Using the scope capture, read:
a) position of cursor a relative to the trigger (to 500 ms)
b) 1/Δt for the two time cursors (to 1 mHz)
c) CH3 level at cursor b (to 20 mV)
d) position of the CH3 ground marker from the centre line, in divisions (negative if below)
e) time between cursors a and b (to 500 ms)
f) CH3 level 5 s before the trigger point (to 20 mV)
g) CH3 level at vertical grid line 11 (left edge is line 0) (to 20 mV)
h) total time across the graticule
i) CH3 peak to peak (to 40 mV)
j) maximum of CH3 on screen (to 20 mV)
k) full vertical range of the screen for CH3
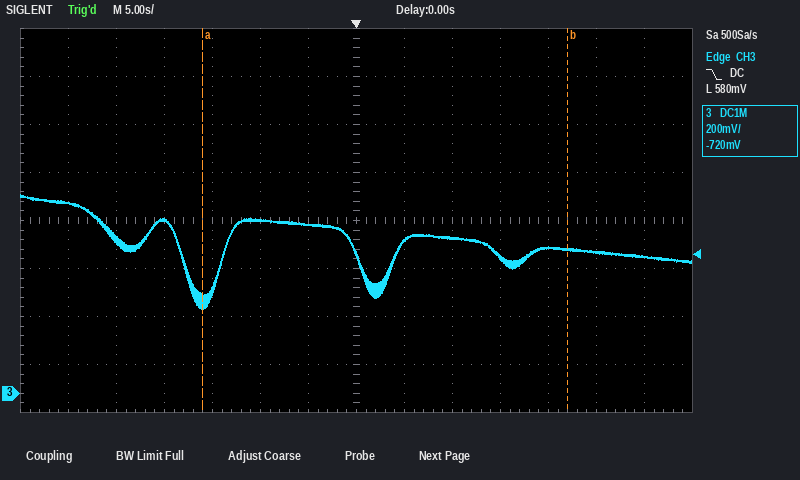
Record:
-16.0 s
26 mHz
600 mV
-3.6 div
38.0 s
700 mV
600 mV
70 s
480 mV
820 mV
1.6 V
